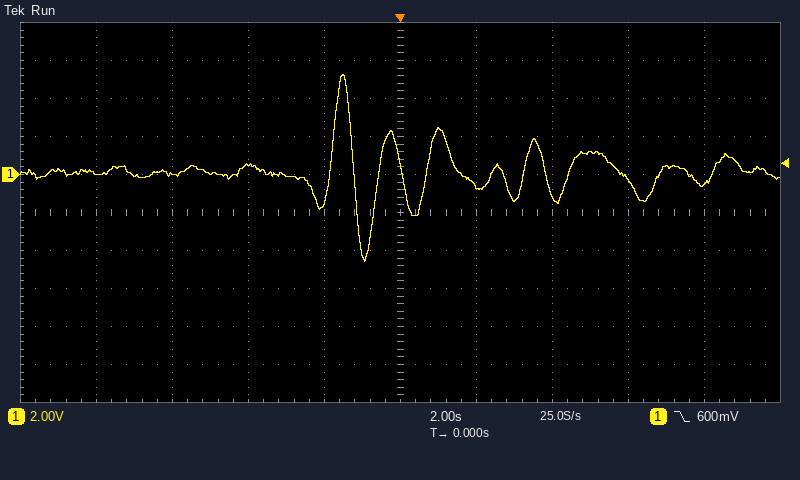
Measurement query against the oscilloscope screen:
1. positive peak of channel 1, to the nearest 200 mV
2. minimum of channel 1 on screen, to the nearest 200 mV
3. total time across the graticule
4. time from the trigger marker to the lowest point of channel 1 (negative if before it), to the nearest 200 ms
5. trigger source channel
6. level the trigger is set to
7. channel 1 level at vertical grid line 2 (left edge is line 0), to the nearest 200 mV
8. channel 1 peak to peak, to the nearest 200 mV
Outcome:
5.2 V
-4.6 V
20 s
-1.0 s
channel 1
600 mV
0.0 V
9.8 V
